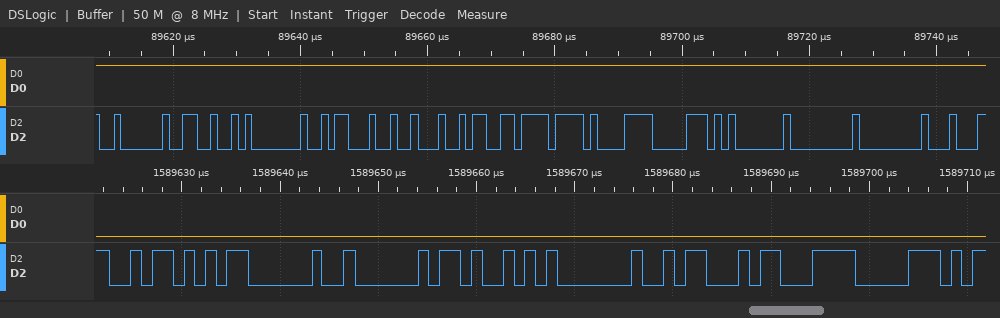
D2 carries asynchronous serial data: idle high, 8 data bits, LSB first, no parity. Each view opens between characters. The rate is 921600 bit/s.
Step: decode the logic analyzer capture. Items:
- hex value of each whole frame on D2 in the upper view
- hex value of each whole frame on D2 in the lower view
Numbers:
02, 26, 01, 1A, 12, 9A, EF, E1, 70, 01, 00, 00
5A, 03, 02, 4B, 01, 1A, E3, 70
